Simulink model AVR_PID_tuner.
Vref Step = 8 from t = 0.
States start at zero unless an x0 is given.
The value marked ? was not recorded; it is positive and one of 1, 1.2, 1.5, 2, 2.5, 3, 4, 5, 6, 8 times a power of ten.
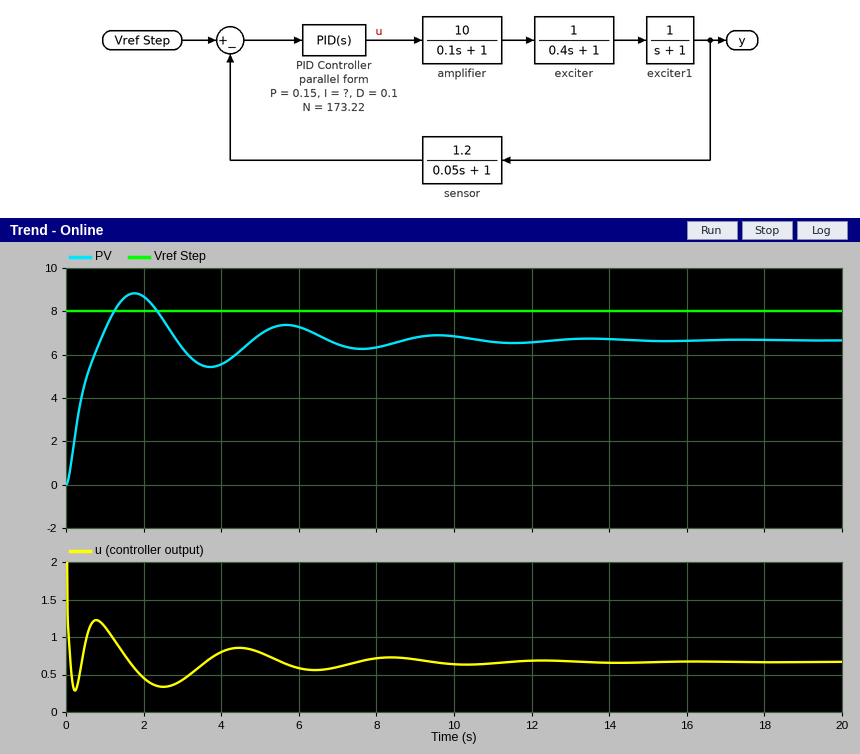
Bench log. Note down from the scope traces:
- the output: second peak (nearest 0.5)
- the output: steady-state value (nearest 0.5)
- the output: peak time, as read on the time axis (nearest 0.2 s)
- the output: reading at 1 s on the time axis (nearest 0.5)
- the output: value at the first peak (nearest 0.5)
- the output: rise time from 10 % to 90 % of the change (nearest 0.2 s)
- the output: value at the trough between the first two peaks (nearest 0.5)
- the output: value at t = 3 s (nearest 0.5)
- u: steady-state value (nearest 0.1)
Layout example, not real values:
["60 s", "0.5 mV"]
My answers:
["7.5", "6.5", "1.8 s", "7.0", "9.0", "0.6 s", "5.5", "6.5", "0.7"]
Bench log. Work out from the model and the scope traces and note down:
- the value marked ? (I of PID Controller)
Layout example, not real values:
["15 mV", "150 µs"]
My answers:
["0.5"]
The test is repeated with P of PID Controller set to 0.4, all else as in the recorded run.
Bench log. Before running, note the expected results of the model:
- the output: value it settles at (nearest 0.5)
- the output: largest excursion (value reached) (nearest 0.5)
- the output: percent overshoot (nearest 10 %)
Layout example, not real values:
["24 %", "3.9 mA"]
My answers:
["6.5", "8.0", "20 %"]
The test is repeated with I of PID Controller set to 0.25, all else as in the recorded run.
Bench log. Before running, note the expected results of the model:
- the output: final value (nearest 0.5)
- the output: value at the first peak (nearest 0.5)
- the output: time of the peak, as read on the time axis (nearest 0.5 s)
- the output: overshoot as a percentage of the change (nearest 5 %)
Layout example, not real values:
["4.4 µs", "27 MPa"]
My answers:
["6.5", "7.5", "2.5 s", "15 %"]
